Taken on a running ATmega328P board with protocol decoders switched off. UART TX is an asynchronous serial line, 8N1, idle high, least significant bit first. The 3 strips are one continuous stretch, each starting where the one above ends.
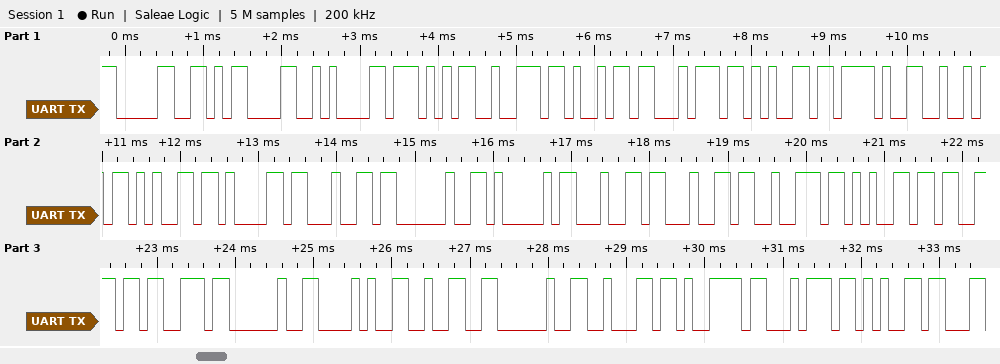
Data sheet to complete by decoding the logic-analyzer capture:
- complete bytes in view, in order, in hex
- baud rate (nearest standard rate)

0x30 0x0D 0x0A 0x57 0x72 0x69 0x74 0x65 0x2F 0x52 0x65 0x61 0x64 0x20 0x41 0x64 0x64 0x72 0x65 0x73 0x73 0x20 0x28 0x32 0x20 0x62 0x79 0x74 0x65
9600 baud
